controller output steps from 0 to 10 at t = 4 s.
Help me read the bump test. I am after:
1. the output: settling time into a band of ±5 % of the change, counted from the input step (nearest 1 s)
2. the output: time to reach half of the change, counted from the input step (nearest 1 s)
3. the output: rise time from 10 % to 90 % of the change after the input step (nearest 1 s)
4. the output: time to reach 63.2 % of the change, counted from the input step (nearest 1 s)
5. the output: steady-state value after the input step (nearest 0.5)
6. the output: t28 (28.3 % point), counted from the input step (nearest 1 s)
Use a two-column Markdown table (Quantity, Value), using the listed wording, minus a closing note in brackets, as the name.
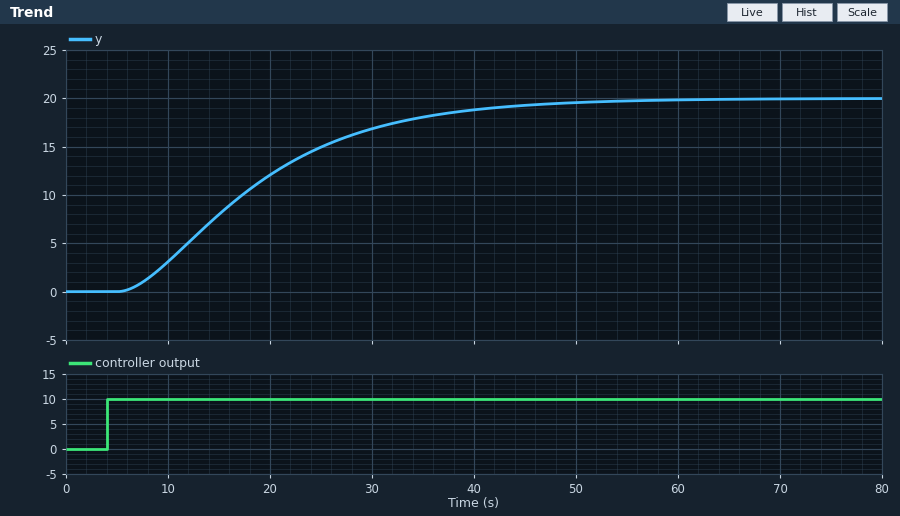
| Quantity | Value |
|---|---|
| the output: settling time into a band of ±5 % of the change, counted from the input step | 38 s |
| the output: time to reach half of the change, counted from the input step | 13 s |
| the output: rise time from 10 % to 90 % of the change after the input step | 26 s |
| the output: time to reach 63.2 % of the change, counted from the input step | 17 s |
| the output: steady-state value after the input step | 20.0 |
| the output: t28 (28.3 % point), counted from the input step | 9 s |
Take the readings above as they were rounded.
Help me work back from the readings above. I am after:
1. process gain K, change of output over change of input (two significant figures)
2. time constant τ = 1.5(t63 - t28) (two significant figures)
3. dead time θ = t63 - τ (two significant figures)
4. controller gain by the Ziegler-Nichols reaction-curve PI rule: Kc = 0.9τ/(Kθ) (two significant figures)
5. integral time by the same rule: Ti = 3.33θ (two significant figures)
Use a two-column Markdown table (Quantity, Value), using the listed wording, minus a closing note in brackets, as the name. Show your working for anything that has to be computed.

| Quantity | Value |
|---|---|
| process gain K, change of output over change of input | (20 - 0) / 10 = 2.0 |
| time constant τ = 1.5(t63 - t28) | 1.5 × (17 - 9) = 12 s |
| dead time θ = t63 - τ | 17 - 12 = 5.0 s |
| controller gain by the Ziegler-Nichols reaction-curve PI rule: Kc = 0.9τ/(Kθ) | 0.9 × 12 / (2 × 5) = 1.1 |
| integral time by the same rule: Ti = 3.33θ | 3.33 × 5 = 17 s |
